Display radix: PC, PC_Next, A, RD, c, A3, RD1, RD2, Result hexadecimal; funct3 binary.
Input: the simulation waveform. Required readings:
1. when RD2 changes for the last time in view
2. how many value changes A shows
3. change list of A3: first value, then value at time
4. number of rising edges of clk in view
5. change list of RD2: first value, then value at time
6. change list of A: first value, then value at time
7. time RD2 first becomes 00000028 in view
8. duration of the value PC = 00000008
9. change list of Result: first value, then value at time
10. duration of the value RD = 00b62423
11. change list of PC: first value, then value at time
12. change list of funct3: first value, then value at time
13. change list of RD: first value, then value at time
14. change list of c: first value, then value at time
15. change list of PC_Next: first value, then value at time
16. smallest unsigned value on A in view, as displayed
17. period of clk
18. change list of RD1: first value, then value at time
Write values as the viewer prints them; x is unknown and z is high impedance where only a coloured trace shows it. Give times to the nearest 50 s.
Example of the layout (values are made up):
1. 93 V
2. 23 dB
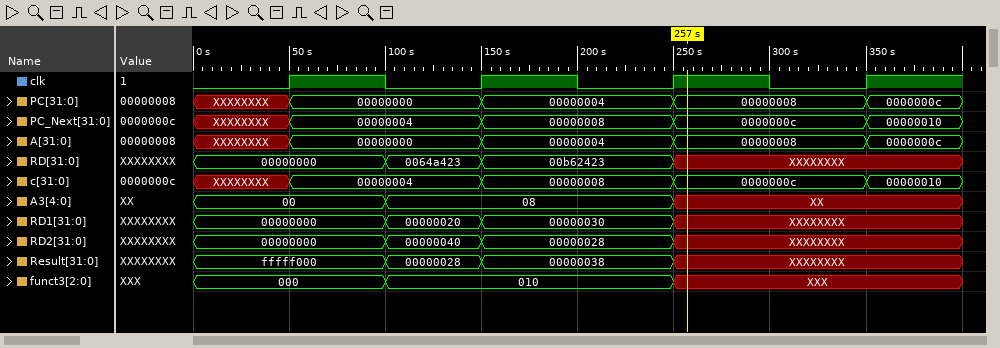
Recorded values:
1. 250 s
2. 4
3. 00, 08 at 100 s, XX at 250 s
4. 4
5. 00000000, 00000040 at 100 s, 00000028 at 150 s, XXXXXXXX at 250 s
6. XXXXXXXX, 00000000 at 50 s, 00000004 at 150 s, 00000008 at 250 s, 0000000c at 350 s
7. 150 s
8. 100 s
9. fffff000, 00000028 at 100 s, 00000038 at 150 s, XXXXXXXX at 250 s
10. 100 s
11. XXXXXXXX, 00000000 at 50 s, 00000004 at 150 s, 00000008 at 250 s, 0000000c at 350 s
12. 000, 010 at 100 s, XXX at 250 s
13. 00000000, 0064a423 at 100 s, 00b62423 at 150 s, XXXXXXXX at 250 s
14. XXXXXXXX, 00000004 at 50 s, 00000008 at 150 s, 0000000c at 250 s, 00000010 at 350 s
15. XXXXXXXX, 00000004 at 50 s, 00000008 at 150 s, 0000000c at 250 s, 00000010 at 350 s
16. 00000000
17. 100 s
18. 00000000, 00000020 at 100 s, 00000030 at 150 s, XXXXXXXX at 250 s
